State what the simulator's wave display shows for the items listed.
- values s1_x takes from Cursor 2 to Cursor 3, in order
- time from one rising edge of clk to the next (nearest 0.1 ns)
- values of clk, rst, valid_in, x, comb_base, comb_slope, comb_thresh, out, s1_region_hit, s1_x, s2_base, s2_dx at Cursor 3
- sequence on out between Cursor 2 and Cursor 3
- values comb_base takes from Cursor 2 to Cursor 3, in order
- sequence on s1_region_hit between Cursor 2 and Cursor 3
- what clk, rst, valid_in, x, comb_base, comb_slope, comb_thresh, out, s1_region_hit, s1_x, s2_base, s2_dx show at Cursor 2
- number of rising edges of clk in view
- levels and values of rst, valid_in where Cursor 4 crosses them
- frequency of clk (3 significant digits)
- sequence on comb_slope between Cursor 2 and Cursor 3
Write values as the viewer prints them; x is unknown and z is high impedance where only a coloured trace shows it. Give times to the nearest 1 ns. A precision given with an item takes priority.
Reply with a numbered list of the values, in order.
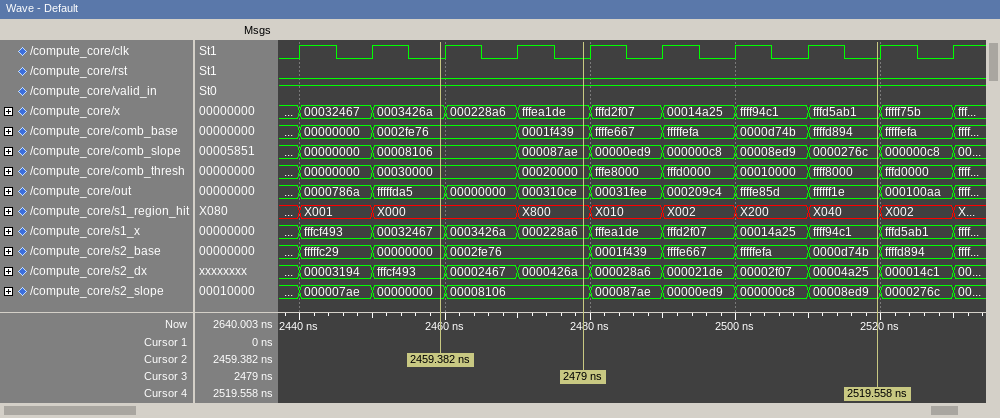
1. 00032467, 0003426a, 000228a6
2. 10 ns
3. clk=0, rst=0, valid_in=1, x=fffea1de, comb_base=0001f439, comb_slope=000087ae, comb_thresh=00020000, out=000310ce, s1_region_hit=X800, s1_x=000228a6, s2_base=0002fe76, s2_dx=0000426a
4. fffffda5, 00000000, 000310ce
5. 0002fe76, 0001f439
6. X000, X800
7. clk=0, rst=0, valid_in=1, x=0003426a, comb_base=0002fe76, comb_slope=00008106, comb_thresh=00030000, out=fffffda5, s1_region_hit=X000, s1_x=00032467, s2_base=00000000, s2_dx=fffcf493
8. 10
9. rst=0, valid_in=1
10. 100 MHz
11. 00008106, 000087ae
